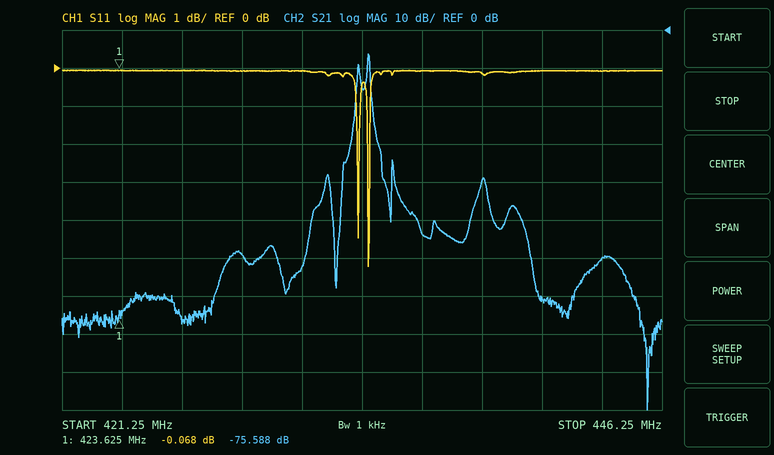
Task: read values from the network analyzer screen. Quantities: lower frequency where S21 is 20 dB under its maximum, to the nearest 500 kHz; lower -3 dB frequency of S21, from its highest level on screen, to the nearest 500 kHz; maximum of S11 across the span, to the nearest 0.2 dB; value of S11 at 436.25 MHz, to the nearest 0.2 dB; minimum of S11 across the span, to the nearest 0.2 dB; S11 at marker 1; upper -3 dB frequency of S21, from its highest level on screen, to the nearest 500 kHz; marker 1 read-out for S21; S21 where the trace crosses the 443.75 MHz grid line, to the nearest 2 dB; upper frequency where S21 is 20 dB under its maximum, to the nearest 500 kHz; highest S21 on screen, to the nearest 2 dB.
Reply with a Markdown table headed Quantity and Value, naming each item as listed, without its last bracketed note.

| Quantity | Value |
|---|---|
| lower frequency where S21 is 20 dB under its maximum, to the nearest 500 kHz | 433.5 MHz |
| lower -3 dB frequency of S21, from its highest level on screen, to the nearest 500 kHz | 434.0 MHz |
| maximum of S11 across the span, to the nearest 0.2 dB | 0.0 dB |
| value of S11 at 436.25 MHz, to the nearest 0.2 dB | 0.0 dB |
| minimum of S11 across the span, to the nearest 0.2 dB | -5.2 dB |
| S11 at marker 1 | -0.068 dB |
| upper -3 dB frequency of S21, from its highest level on screen, to the nearest 500 kHz | 434.0 MHz |
| marker 1 read-out for S21 | -75.588 dB |
| S21 where the trace crosses the 443.75 MHz grid line, to the nearest 2 dB | -60 dB |
| upper frequency where S21 is 20 dB under its maximum, to the nearest 500 kHz | 434.5 MHz |
| highest S21 on screen, to the nearest 2 dB | -6 dB |
